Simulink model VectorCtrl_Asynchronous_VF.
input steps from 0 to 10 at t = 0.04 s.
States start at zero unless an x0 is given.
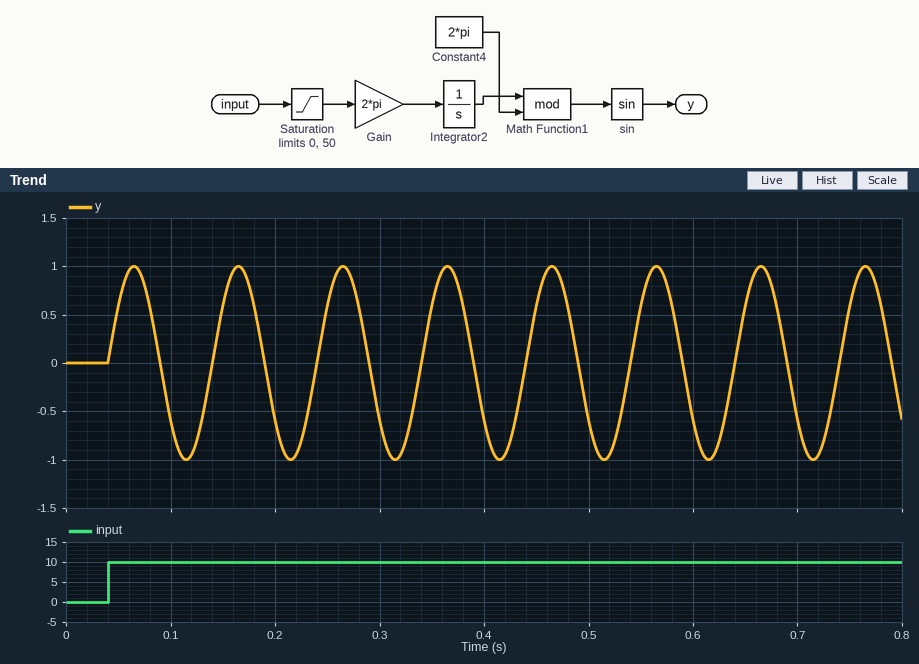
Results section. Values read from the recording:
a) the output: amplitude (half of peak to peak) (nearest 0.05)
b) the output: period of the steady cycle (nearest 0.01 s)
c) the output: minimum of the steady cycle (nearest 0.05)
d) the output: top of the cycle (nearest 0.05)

1.00
0.10 s
-1.00
1.00
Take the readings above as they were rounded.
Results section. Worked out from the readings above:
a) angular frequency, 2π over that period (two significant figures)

63 rad/s
